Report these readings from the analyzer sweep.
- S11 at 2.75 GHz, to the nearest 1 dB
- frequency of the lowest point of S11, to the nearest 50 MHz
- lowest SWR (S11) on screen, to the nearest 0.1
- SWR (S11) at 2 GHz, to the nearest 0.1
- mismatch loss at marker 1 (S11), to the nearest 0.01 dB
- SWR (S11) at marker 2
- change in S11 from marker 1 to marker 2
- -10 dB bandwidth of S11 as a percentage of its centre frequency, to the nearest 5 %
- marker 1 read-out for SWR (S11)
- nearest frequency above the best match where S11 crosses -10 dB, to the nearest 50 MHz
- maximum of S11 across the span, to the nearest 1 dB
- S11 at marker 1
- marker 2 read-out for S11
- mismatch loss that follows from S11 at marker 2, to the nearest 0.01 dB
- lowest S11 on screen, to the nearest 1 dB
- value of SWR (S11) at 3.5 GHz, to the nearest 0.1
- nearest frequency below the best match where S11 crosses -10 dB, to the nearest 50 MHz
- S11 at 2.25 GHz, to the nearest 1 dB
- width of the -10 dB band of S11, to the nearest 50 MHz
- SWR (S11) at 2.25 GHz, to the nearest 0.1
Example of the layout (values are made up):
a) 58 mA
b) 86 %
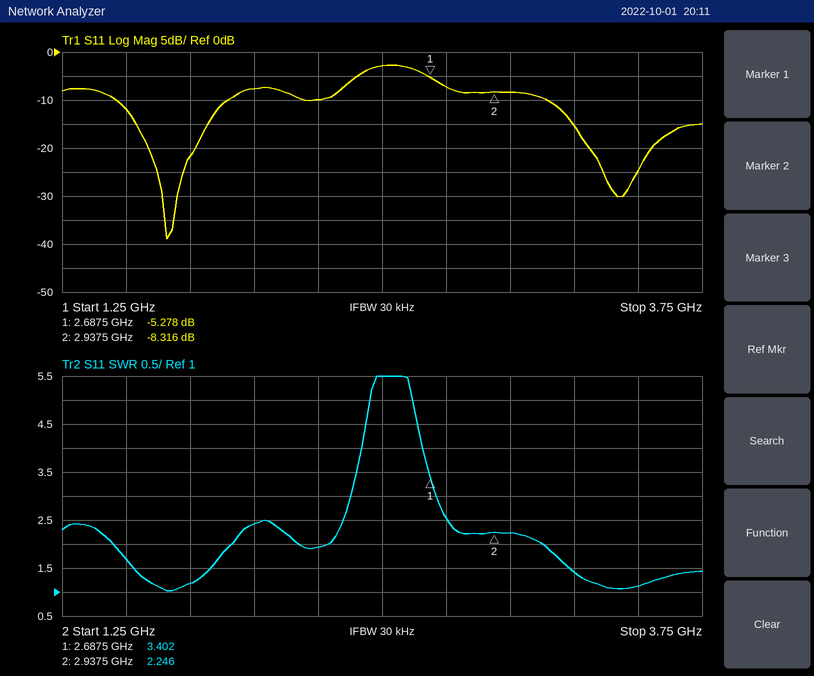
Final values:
a) -7 dB
b) 1.65 GHz
c) 1.0
d) 2.4
e) 1.53 dB
f) 2.246
g) -3.038 dB
h) 25 %
i) 3.402
j) 1.90 GHz
k) -3 dB
l) -5.278 dB
m) -8.316 dB
n) 0.69 dB
o) -39 dB
p) 1.1
q) 1.45 GHz
r) -10 dB
s) 450 MHz
t) 1.9
